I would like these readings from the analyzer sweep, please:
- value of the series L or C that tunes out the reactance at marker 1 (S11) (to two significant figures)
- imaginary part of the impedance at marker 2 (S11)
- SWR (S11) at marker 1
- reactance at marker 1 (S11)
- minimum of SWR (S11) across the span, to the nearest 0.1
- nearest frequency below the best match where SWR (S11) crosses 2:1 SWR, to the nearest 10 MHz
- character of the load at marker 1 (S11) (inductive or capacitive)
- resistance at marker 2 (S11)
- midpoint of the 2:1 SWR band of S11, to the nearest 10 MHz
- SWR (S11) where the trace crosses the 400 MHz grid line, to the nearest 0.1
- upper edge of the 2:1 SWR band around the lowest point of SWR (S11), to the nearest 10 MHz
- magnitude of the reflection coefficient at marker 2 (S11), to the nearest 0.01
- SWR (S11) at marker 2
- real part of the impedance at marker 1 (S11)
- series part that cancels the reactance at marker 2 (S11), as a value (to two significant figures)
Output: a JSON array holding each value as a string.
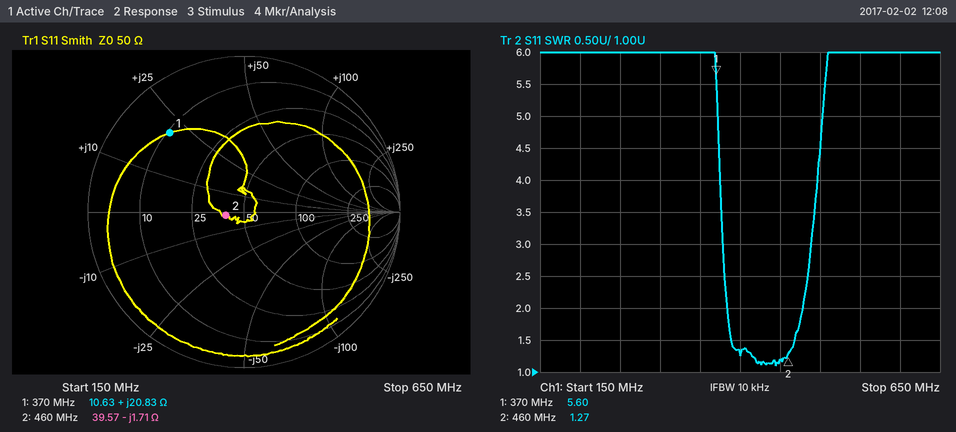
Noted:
["21 pF", "-1.71 Ω", "5.60", "+20.83 Ω", "1.1", "380 MHz", "inductive", "39.57 Ω", "430 MHz", "1.3", "480 MHz", "0.12", "1.27", "10.63 Ω", "590 pH"]
